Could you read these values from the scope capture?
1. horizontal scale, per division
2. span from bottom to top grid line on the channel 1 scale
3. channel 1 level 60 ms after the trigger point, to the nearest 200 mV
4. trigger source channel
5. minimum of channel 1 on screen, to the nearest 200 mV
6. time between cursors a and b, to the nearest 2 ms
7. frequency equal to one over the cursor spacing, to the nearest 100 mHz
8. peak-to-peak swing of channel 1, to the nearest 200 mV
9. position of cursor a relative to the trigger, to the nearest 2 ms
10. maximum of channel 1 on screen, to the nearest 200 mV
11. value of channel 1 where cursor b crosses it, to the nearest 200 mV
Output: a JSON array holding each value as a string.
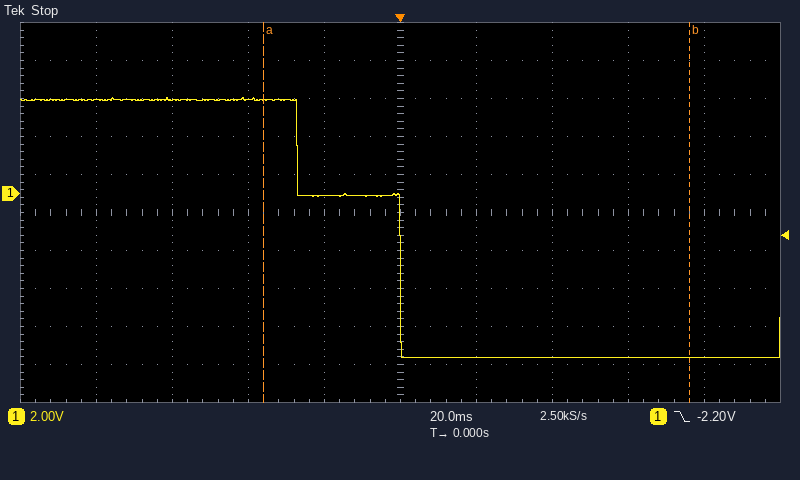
["20 ms", "20 V", "-8.6 V", "channel 1", "-8.6 V", "112 ms", "8.9 Hz", "13.6 V", "-36 ms", "5.0 V", "-8.6 V"]
